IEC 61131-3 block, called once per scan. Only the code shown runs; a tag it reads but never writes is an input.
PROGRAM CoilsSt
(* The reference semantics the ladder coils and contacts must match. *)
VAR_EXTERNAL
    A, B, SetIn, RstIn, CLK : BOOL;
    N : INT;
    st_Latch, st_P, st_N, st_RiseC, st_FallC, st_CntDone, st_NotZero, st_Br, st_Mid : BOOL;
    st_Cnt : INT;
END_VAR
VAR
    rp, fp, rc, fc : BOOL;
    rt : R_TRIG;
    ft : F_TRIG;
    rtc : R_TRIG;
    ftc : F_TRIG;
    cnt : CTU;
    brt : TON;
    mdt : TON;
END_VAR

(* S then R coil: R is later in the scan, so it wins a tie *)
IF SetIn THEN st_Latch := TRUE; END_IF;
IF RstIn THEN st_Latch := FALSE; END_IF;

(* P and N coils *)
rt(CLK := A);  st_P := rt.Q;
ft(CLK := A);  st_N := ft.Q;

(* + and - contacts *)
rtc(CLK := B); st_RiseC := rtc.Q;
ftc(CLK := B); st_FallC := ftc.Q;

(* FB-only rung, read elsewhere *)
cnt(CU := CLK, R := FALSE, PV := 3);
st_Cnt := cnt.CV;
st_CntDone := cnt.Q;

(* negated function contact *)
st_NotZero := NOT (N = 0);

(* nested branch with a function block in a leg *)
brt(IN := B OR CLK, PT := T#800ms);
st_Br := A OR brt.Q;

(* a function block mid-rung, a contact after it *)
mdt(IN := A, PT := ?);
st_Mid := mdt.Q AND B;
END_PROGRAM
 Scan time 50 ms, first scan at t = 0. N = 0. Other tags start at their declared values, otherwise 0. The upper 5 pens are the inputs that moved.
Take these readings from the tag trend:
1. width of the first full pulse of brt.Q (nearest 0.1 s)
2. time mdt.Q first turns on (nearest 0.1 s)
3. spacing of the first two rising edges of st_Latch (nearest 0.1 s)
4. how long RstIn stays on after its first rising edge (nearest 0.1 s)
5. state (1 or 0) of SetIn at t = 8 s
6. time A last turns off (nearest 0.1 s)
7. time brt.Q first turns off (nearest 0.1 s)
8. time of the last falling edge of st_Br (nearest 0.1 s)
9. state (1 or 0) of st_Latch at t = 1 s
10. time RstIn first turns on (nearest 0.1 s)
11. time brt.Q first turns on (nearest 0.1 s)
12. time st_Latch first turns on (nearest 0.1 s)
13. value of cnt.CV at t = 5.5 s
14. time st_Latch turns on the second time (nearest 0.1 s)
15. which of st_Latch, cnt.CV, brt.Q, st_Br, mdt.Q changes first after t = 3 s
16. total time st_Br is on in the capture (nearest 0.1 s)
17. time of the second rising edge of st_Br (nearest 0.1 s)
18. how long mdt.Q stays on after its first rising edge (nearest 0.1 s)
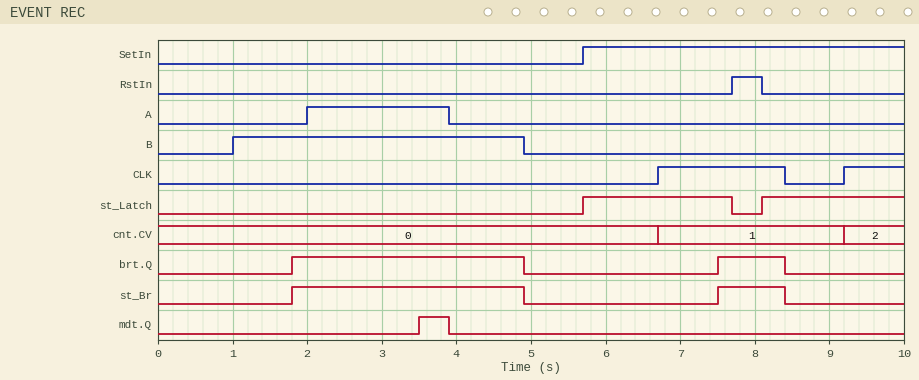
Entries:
3.1 s
3.5 s
2.4 s
0.4 s
1
3.9 s
4.9 s
8.4 s
0
7.7 s
1.8 s
5.7 s
0
8.1 s
mdt.Q
4.0 s
7.5 s
0.4 s
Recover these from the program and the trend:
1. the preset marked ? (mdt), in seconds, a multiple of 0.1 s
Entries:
1.5 s
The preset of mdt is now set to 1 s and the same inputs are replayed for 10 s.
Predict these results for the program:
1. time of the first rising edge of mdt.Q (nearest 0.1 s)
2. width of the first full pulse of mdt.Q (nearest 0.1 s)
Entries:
3.0 s
0.9 s
